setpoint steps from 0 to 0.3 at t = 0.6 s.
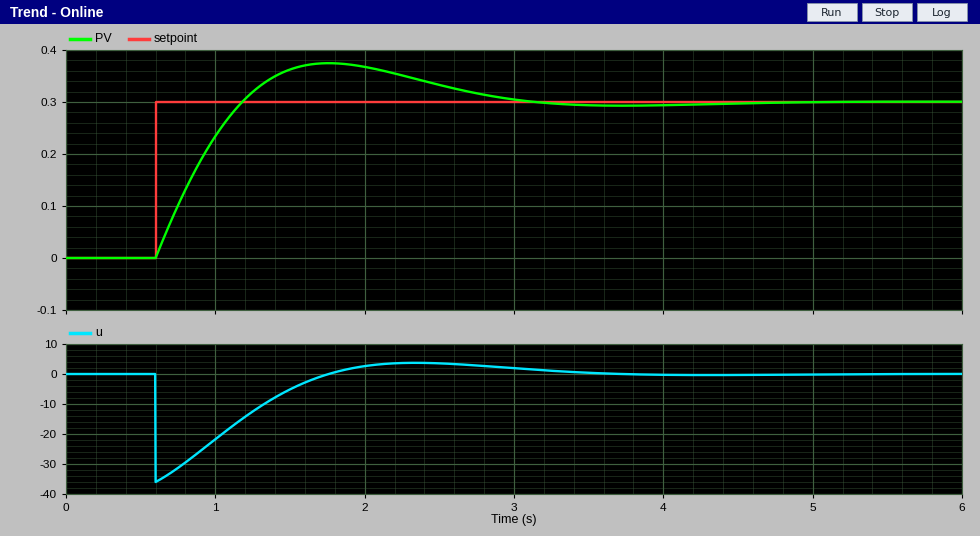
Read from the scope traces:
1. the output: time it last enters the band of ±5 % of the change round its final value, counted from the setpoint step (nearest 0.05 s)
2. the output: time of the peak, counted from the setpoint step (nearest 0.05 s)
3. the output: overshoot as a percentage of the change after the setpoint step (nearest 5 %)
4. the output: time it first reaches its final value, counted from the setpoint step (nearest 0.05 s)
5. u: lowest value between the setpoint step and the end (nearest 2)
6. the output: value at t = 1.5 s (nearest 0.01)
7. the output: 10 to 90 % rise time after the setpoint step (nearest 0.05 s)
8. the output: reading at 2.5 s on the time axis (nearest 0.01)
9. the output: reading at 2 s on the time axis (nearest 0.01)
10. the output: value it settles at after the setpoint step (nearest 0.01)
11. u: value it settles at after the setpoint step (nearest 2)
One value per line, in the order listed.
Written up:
2.20 s
1.15 s
25 %
0.60 s
-36
0.36
0.45 s
0.33
0.37
0.30
0
